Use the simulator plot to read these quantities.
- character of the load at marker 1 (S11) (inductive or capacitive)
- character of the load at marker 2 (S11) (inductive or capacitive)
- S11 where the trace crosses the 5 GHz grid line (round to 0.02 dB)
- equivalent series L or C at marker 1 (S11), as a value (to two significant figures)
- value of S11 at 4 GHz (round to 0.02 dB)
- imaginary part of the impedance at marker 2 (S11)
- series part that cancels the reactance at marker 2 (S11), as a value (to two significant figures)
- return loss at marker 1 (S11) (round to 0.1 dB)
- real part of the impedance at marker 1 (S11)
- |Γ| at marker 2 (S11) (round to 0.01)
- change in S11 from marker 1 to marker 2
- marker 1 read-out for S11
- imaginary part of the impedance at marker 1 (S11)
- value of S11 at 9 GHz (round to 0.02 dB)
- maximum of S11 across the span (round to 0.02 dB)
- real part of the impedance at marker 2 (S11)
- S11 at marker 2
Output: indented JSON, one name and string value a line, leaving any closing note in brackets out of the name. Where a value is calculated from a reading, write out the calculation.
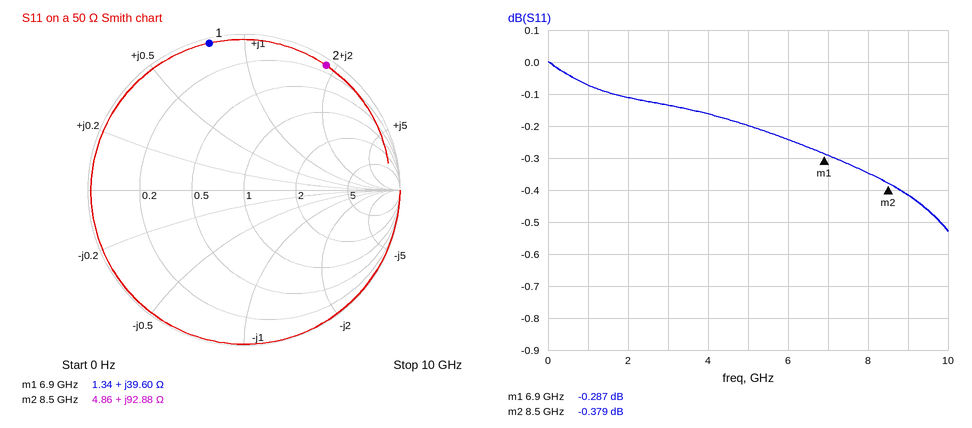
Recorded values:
{
  "character of the load at marker 1 (S11)": "inductive",
  "character of the load at marker 2 (S11)": "inductive",
  "S11 where the trace crosses the 5 GHz grid line": "-0.20 dB",
  "equivalent series L or C at marker 1 (S11), as a value": "L = 39.6 Ω/(2π × 6.9 GHz) ≈ 913 pH, so 910 pH to two significant figures",
  "value of S11 at 4 GHz": "-0.16 dB",
  "imaginary part of the impedance at marker 2": "+92.88 Ω",
  "series part that cancels the reactance at marker 2 (S11), as a value": "C = 1/(2π × 8.5 GHz × 92.88 Ω) ≈ 202 fF, so 200 fF to two significant figures",
  "return loss at marker 1 (S11)": "0.3 dB",
  "real part of the impedance at marker 1": "1.34 Ω",
  "|Γ| at marker 2 (S11)": "0.96",
  "change in S11 from marker 1 to marker 2": "-0.379 − (-0.287) = -0.092 dB",
  "marker 1 read-out for S11": "-0.287 dB",
  "imaginary part of the impedance at marker 1": "+39.60 Ω",
  "value of S11 at 9 GHz": "-0.42 dB",
  "maximum of S11 across the span": "0.00 dB",
  "real part of the impedance at marker 2": "4.86 Ω",
  "S11 at marker 2": "-0.379 dB"
}
